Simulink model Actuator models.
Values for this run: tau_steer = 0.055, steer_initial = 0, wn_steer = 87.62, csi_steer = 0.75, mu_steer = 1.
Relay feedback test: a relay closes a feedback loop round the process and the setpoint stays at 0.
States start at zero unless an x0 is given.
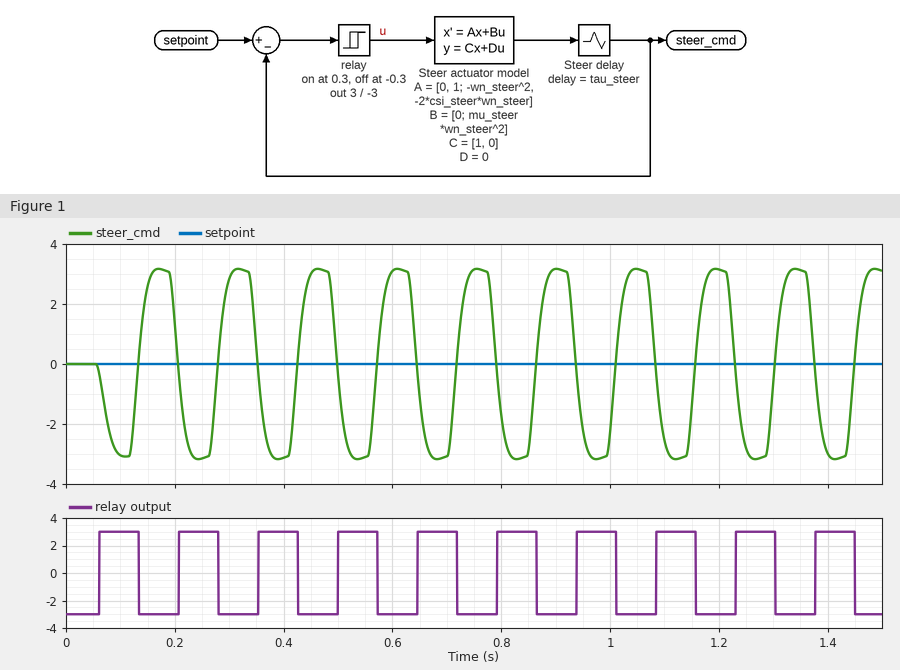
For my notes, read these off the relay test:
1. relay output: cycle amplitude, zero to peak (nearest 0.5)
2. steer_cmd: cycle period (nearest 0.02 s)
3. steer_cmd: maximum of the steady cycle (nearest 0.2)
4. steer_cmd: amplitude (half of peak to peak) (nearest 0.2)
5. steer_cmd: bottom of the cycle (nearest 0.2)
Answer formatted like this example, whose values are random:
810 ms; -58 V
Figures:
3.0; 0.14 s; 3.2; 3.2; -3.2
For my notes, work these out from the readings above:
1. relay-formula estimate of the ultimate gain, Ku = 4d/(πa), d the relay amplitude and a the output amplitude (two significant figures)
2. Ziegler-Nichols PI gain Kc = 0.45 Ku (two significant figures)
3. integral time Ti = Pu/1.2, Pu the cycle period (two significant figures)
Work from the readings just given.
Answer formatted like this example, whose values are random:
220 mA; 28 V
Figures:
1.2; 0.54; 0.12 s
